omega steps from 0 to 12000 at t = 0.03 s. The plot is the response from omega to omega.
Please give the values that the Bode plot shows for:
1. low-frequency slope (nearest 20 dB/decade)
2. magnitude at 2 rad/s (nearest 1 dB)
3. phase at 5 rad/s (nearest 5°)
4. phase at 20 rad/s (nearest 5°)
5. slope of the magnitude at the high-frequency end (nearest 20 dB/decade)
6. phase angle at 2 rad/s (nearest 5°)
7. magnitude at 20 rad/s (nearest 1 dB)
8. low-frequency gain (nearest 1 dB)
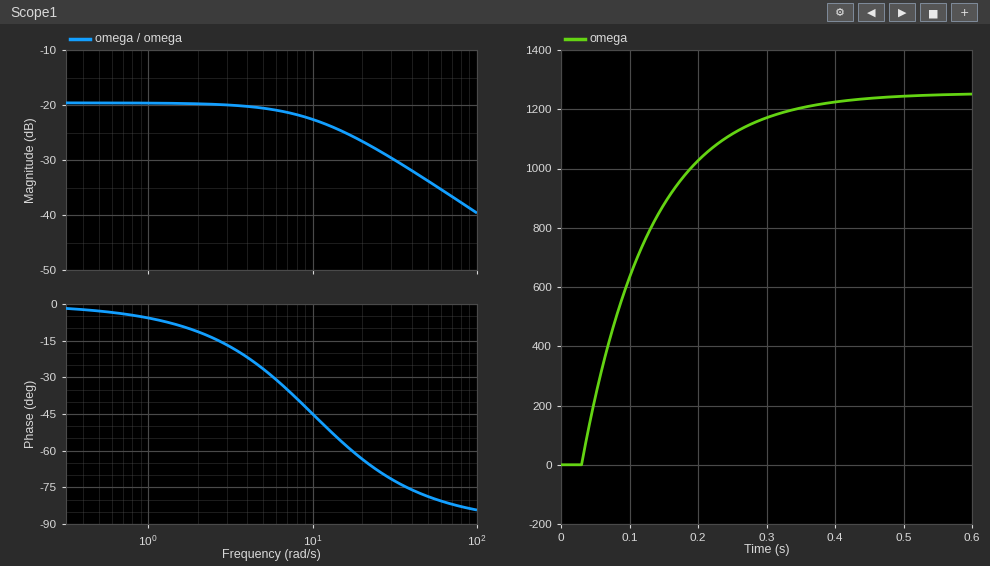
0 dB/decade
-20 dB
-25°
-65°
-20 dB/decade
-10°
-27 dB
-20 dB
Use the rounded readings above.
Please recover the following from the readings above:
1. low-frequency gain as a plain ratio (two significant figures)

0.10
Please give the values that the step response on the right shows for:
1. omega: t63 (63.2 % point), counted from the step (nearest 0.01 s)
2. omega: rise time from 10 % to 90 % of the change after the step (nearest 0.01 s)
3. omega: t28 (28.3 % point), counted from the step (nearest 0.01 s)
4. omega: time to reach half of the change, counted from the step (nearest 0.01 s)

0.10 s
0.22 s
0.03 s
0.07 s
